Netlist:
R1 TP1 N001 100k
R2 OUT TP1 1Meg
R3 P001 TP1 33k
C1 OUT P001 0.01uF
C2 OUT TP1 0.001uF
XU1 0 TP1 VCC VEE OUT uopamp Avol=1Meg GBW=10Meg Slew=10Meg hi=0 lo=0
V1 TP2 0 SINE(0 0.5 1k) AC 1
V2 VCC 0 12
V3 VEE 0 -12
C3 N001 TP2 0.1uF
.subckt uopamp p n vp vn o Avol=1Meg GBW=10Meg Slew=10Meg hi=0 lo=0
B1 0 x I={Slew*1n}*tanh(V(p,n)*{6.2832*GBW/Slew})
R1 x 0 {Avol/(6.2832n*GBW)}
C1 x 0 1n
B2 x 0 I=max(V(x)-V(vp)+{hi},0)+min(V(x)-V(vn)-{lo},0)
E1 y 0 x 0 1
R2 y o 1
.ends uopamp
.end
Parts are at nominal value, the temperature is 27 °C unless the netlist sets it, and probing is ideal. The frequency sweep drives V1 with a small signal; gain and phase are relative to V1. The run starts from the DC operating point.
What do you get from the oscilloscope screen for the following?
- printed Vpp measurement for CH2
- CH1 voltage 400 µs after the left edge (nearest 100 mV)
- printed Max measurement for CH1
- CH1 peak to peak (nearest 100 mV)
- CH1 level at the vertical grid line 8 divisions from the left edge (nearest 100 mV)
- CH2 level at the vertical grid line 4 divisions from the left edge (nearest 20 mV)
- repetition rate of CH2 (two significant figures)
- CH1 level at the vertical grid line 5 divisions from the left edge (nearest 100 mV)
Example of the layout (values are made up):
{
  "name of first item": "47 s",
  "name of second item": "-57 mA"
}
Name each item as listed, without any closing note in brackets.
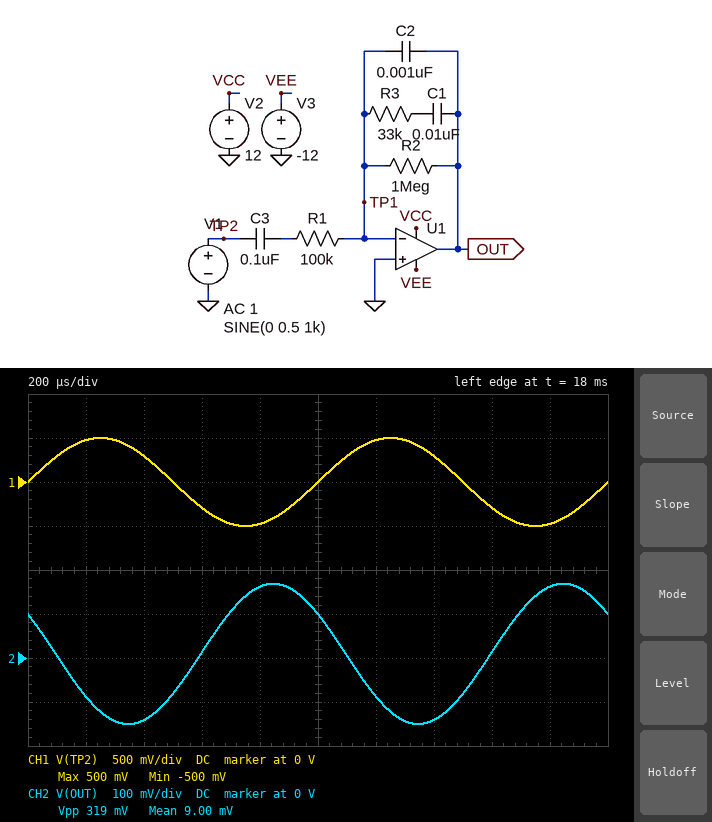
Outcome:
{
  "printed Vpp measurement for CH2": "319 mV",
  "CH1 voltage 400 µs after the left edge": "300 mV",
  "printed Max measurement for CH1": "500 mV",
  "CH1 peak to peak": "1.0 V",
  "CH1 level at the vertical grid line 8 divisions from the left edge": "-300 mV",
  "CH2 level at the vertical grid line 4 divisions from the left edge": "160 mV",
  "repetition rate of CH2": "1.0 kHz",
  "CH1 level at the vertical grid line 5 divisions from the left edge": "0 V"
}
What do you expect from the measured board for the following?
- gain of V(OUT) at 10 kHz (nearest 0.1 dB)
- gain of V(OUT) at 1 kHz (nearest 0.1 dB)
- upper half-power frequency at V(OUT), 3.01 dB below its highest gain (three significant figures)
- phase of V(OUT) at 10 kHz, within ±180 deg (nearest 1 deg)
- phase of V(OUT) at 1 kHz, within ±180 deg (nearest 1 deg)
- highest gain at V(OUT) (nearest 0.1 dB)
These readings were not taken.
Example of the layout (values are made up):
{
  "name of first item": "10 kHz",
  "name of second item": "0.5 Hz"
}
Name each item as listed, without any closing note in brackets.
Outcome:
{
  "gain of V(OUT) at 10 kHz": "-17.1 dB",
  "gain of V(OUT) at 1 kHz": "-9.9 dB",
  "upper half-power frequency at V(OUT), 3.01 dB below its highest gain": "36.3 Hz",
  "phase of V(OUT) at 10 kHz, within ±180 deg": "116 deg",
  "phase of V(OUT) at 1 kHz, within ±180 deg": "146 deg",
  "highest gain at V(OUT)": "13.4 dB"
}
